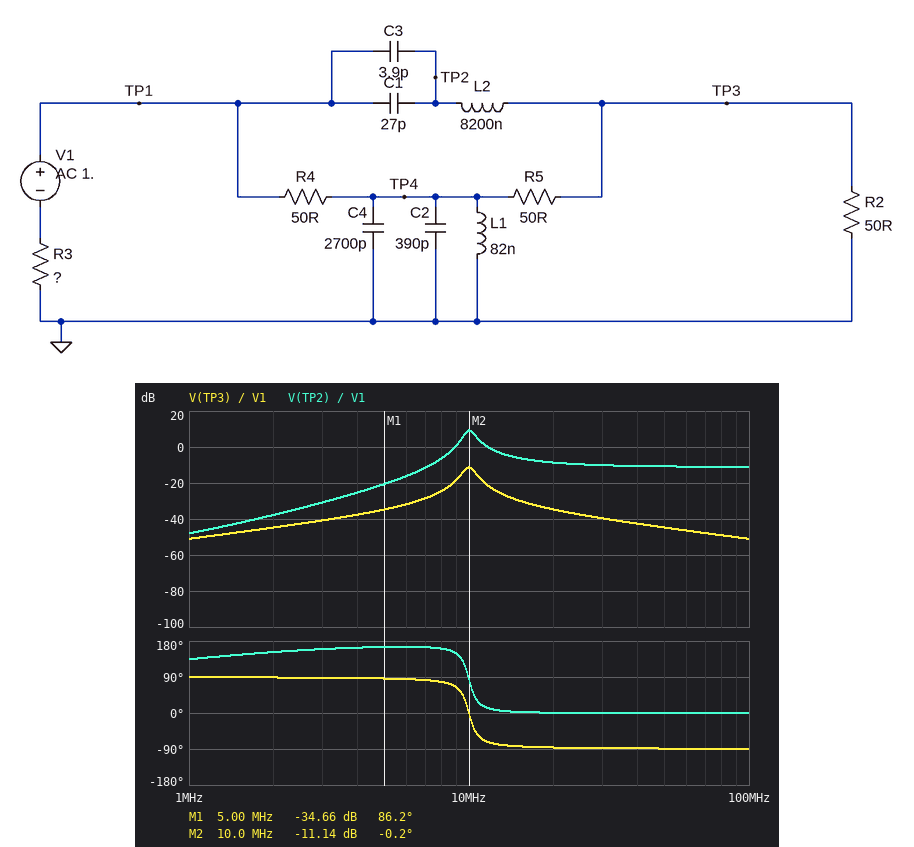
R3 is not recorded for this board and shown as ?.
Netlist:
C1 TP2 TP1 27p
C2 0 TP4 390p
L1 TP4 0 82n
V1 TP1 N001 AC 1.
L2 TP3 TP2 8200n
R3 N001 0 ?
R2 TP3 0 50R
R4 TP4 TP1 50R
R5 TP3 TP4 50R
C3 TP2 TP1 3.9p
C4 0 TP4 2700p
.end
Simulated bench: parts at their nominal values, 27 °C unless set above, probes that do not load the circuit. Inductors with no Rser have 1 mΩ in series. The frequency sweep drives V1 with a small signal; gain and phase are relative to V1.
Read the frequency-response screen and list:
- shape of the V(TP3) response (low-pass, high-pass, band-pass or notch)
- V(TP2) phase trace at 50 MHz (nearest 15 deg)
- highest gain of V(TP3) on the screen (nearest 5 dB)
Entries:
band-pass
0 deg
-10 dB
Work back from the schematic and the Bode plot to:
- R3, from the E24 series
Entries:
130 Ω
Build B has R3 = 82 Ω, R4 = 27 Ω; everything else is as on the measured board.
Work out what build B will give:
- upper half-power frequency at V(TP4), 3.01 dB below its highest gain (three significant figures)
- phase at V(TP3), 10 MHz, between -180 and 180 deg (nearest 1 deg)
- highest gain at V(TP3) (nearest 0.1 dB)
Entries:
10.7 MHz
0 deg
-8.4 dB
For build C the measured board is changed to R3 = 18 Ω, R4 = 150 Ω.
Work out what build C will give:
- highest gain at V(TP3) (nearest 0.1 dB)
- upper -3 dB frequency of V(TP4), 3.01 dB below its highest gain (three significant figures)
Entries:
-2.7 dB
10.4 MHz
